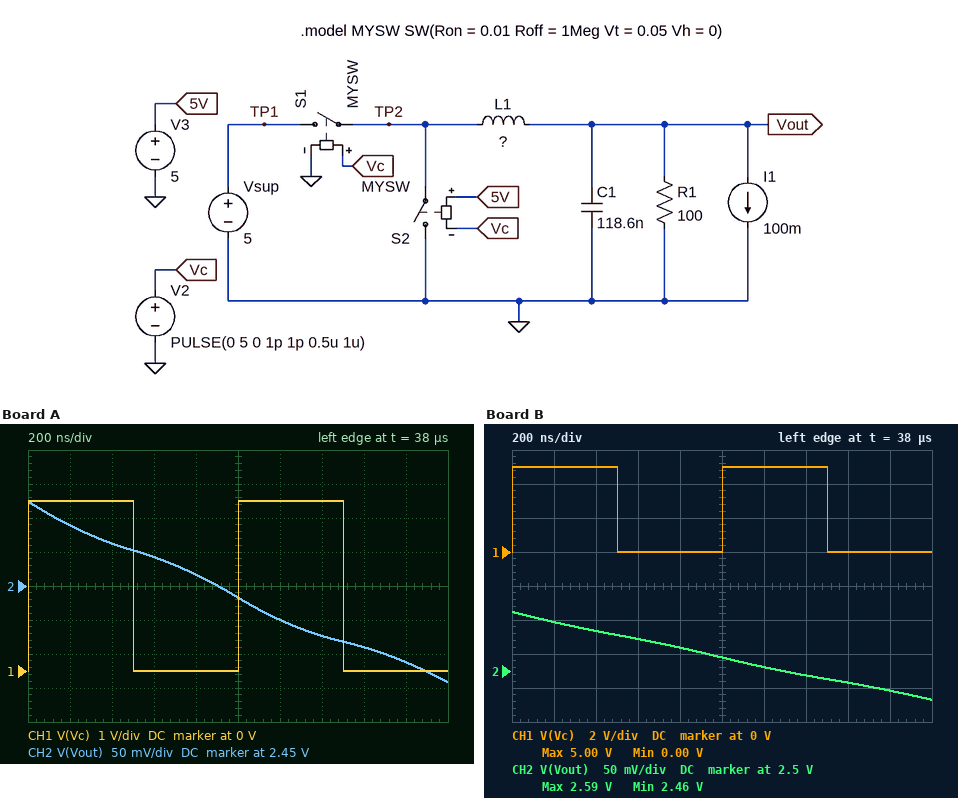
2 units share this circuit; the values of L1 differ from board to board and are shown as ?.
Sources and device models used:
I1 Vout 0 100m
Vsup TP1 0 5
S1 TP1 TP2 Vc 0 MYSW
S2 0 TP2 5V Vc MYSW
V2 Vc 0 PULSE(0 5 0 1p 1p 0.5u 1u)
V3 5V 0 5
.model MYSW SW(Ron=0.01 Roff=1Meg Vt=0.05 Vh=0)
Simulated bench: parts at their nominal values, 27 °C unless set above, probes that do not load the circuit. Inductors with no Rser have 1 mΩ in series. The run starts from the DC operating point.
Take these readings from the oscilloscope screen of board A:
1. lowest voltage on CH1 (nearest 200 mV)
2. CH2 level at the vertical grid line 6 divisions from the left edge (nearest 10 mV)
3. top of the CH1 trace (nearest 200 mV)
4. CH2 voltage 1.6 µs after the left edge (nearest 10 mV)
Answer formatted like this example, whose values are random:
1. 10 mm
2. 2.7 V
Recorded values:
1. 0 V
2. 2.40 V
3. 5.0 V
4. 2.36 V
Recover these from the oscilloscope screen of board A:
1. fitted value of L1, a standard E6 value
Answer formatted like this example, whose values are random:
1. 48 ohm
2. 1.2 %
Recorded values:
1. 100 µH
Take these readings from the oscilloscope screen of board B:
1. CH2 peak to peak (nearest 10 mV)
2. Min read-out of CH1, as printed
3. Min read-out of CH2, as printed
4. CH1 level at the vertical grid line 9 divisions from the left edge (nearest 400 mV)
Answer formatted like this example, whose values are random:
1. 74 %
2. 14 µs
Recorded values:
1. 130 mV
2. 0.00 V
3. 2.46 V
4. 0 V
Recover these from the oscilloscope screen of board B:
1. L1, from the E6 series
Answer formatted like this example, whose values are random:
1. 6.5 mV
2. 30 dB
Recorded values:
1. 470 µH
